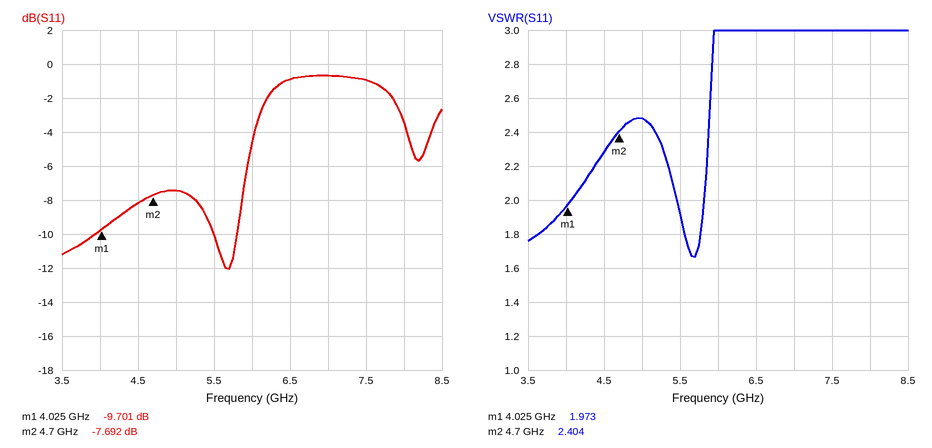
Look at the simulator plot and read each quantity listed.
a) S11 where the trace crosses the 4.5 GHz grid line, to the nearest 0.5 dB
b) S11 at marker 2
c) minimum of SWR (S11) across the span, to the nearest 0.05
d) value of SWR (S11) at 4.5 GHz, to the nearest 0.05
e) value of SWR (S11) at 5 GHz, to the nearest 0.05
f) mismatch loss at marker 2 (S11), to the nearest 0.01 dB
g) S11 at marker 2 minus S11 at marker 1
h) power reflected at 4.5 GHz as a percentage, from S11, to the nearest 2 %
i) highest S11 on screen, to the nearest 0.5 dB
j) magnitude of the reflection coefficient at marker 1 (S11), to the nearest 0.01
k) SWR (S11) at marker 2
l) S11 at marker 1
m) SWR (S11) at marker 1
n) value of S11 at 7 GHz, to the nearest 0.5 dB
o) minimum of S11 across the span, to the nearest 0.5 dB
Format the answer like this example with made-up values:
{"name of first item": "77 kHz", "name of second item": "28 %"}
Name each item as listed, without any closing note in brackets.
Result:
{"S11 where the trace crosses the 4.5 GHz grid line, to the nearest 0.5 dB": "-8.0 dB", "S11 at marker 2": "-7.692 dB", "minimum of SWR (S11) across the span, to the nearest 0.05": "1.65", "value of SWR (S11) at 4.5 GHz, to the nearest 0.05": "2.30", "value of SWR (S11) at 5 GHz, to the nearest 0.05": "2.50", "mismatch loss at marker 2 (S11), to the nearest 0.01 dB": "0.81 dB", "S11 at marker 2 minus S11 at marker 1": "2.009 dB", "power reflected at 4.5 GHz as a percentage, from S11, to the nearest 2 %": "16 %", "highest S11 on screen, to the nearest 0.5 dB": "-0.5 dB", "magnitude of the reflection coefficient at marker 1 (S11), to the nearest 0.01": "0.33", "SWR (S11) at marker 2": "2.404", "S11 at marker 1": "-9.701 dB", "SWR (S11) at marker 1": "1.973", "value of S11 at 7 GHz, to the nearest 0.5 dB": "-0.5 dB", "minimum of S11 across the span, to the nearest 0.5 dB": "-12.0 dB"}
